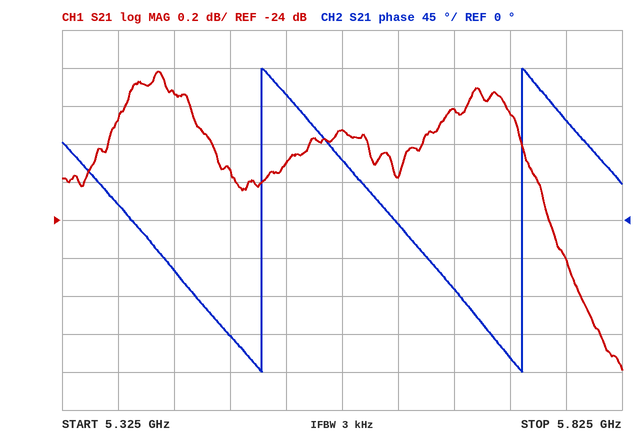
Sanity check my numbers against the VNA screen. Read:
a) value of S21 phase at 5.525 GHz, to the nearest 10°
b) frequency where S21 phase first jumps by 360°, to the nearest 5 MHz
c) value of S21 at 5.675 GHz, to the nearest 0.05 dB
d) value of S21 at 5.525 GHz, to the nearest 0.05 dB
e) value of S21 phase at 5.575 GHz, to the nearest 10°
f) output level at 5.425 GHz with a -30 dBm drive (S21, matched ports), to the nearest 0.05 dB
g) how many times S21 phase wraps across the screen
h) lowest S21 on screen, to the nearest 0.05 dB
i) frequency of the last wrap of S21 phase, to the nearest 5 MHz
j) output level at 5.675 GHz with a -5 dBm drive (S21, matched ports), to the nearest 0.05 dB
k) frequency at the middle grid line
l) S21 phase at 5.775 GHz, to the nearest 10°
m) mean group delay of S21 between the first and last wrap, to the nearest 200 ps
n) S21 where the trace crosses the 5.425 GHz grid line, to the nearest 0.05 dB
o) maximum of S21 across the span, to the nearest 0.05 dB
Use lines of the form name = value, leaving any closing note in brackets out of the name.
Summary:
value of S21 phase at 5.525 GHz, to the nearest 10° = 150°
frequency where S21 phase first jumps by 360°, to the nearest 5 MHz = 5.505 GHz
value of S21 at 5.675 GHz, to the nearest 0.05 dB = -23.40 dB
value of S21 at 5.525 GHz, to the nearest 0.05 dB = -23.70 dB
value of S21 phase at 5.575 GHz, to the nearest 10° = 70°
output level at 5.425 GHz with a -30 dBm drive (S21, matched ports), to the nearest 0.05 dB = -53.35 dBm
how many times S21 phase wraps across the screen = 2
lowest S21 on screen, to the nearest 0.05 dB = -24.80 dB
frequency of the last wrap of S21 phase, to the nearest 5 MHz = 5.735 GHz
output level at 5.675 GHz with a -5 dBm drive (S21, matched ports), to the nearest 0.05 dB = -28.40 dBm
frequency at the middle grid line = 5.575 GHz
S21 phase at 5.775 GHz, to the nearest 10° = 120°
mean group delay of S21 between the first and last wrap, to the nearest 200 ps = 4.4 ns
S21 where the trace crosses the 5.425 GHz grid line, to the nearest 0.05 dB = -23.35 dB
maximum of S21 across the span, to the nearest 0.05 dB = -23.20 dB
